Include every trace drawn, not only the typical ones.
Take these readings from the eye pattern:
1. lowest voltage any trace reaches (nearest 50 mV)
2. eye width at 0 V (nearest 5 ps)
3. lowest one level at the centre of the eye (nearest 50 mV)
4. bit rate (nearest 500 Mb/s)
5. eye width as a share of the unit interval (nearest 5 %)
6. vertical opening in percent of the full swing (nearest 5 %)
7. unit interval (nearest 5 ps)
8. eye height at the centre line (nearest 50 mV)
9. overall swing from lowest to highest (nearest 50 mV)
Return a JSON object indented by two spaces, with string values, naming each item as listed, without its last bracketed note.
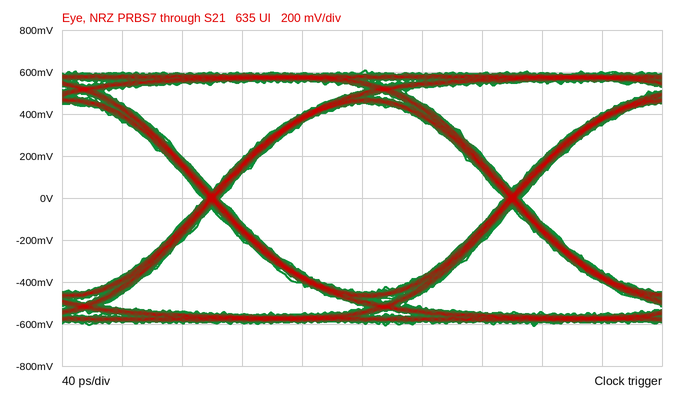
{
  "lowest voltage any trace reaches": "-600 mV",
  "eye width at 0 V": "190 ps",
  "lowest one level at the centre of the eye": "450 mV",
  "bit rate": "5.0 Gb/s",
  "eye width as a share of the unit interval": "95 %",
  "vertical opening in percent of the full swing": "75 %",
  "unit interval": "200 ps",
  "eye height at the centre line": "900 mV",
  "overall swing from lowest to highest": "1.20 V"
}
